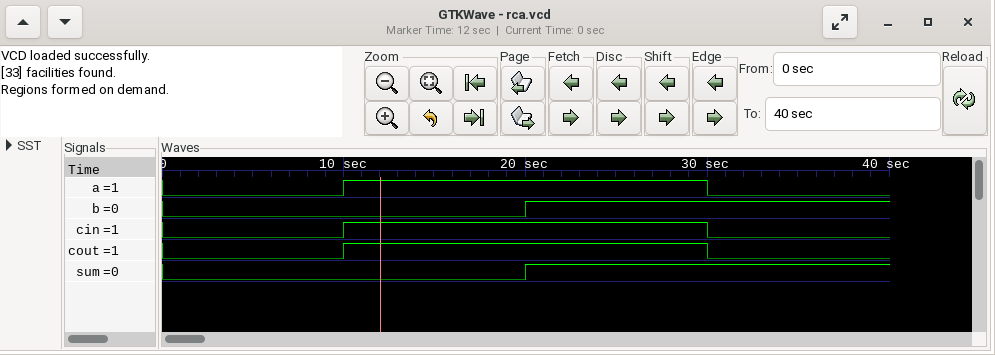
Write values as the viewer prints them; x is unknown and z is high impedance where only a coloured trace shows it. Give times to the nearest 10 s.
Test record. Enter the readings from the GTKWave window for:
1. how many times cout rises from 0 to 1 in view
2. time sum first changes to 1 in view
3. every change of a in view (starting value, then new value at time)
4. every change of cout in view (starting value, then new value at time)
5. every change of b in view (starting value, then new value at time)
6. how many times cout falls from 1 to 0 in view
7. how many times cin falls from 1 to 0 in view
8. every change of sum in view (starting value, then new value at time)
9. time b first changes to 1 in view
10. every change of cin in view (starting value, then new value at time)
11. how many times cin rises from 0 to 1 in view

1
20 s
0, 1 at 10 s, 0 at 30 s
0, 1 at 10 s, 0 at 30 s
0, 1 at 20 s
1
1
0, 1 at 20 s
20 s
0, 1 at 10 s, 0 at 30 s
1
